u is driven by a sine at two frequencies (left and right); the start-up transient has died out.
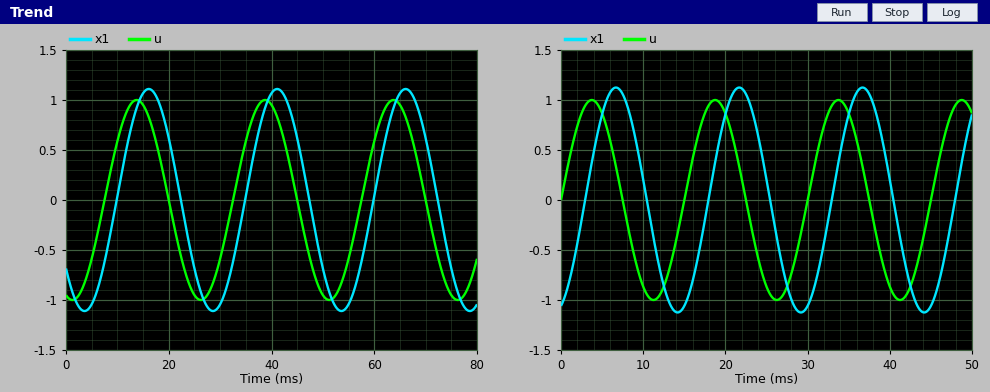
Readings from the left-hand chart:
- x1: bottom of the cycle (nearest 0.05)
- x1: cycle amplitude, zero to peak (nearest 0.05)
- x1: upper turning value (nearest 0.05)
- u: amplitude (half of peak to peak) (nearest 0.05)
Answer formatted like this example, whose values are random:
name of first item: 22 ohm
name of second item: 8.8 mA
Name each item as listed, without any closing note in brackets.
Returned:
x1: bottom of the cycle: -1.10
x1: cycle amplitude, zero to peak: 1.10
x1: upper turning value: 1.10
u: amplitude (half of peak to peak): 1.00
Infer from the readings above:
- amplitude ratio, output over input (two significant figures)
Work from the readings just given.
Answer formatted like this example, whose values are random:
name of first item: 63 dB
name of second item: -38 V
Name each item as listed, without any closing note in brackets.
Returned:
amplitude ratio, output over input: 1.1
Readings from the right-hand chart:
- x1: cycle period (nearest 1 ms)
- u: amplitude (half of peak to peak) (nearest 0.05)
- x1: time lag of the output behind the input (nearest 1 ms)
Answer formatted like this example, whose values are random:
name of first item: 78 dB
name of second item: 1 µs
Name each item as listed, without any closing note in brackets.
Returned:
x1: cycle period: 15 ms
u: amplitude (half of peak to peak): 1.00
x1: time lag of the output behind the input: 3 ms
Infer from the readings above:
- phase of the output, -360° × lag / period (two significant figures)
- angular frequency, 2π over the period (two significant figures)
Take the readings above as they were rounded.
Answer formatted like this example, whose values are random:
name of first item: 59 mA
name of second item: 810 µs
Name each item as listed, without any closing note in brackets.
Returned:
phase of the output, -360° × lag / period: -72°
angular frequency, 2π over the period: 0.42 rad/ms
